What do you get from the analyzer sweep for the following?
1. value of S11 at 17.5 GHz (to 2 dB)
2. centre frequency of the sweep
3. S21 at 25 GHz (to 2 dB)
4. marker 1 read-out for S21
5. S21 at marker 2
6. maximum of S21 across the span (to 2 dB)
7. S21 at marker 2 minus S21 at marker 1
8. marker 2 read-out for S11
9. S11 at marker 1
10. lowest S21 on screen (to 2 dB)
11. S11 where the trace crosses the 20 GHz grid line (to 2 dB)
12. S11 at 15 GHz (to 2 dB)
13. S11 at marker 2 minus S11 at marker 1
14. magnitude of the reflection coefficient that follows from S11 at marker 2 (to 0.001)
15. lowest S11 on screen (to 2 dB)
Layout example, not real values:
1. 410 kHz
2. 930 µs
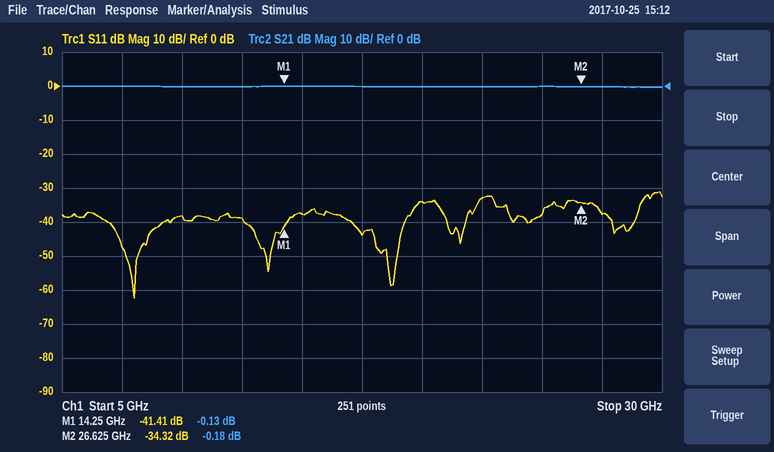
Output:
1. -44 dB
2. 17.5 GHz
3. 0 dB
4. -0.13 dB
5. -0.18 dB
6. 0 dB
7. -0.05 dB
8. -34.32 dB
9. -41.41 dB
10. 0 dB
11. -34 dB
12. -38 dB
13. 7.09 dB
14. 0.019
15. -62 dB
